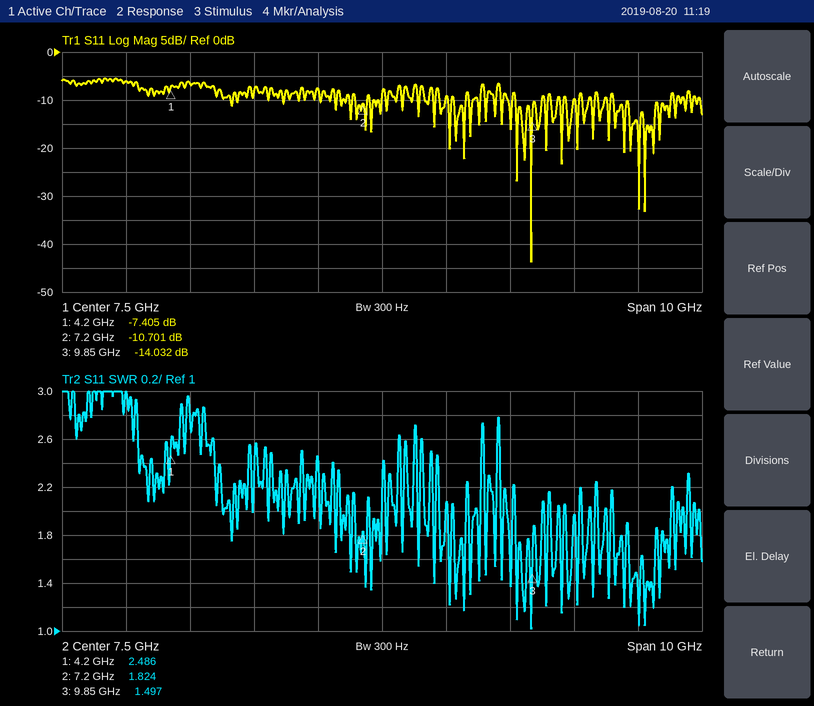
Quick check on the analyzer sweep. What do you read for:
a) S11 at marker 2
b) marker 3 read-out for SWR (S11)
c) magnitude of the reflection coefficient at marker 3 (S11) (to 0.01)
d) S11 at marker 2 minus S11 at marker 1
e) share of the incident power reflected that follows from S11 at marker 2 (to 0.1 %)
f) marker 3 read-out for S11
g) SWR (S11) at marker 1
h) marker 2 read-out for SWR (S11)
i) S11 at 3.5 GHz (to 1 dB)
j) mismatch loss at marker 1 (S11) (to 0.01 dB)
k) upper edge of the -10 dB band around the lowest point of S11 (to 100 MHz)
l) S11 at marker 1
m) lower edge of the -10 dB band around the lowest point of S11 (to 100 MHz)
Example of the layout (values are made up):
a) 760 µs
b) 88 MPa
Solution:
a) -10.701 dB
b) 1.497
c) 0.20
d) -3.296 dB
e) 8.5 %
f) -14.032 dB
g) 2.486
h) 1.824
i) -6 dB
j) 0.87 dB
k) 10.0 GHz
l) -7.405 dB
m) 9.6 GHz
